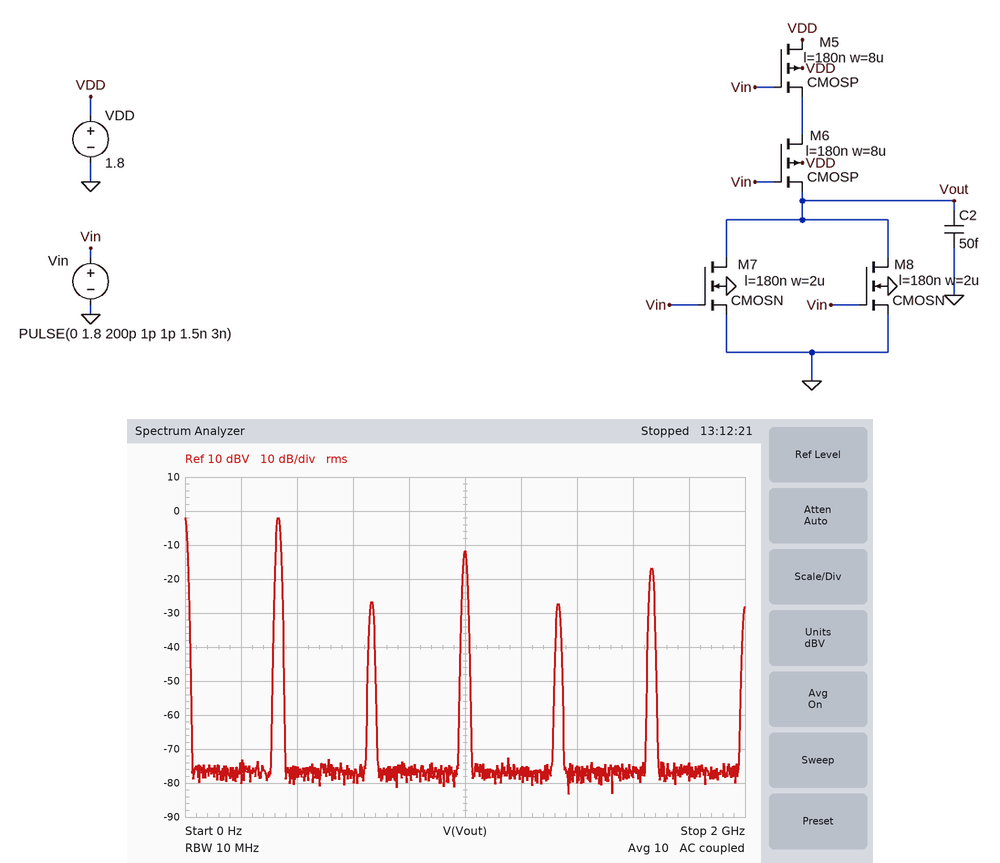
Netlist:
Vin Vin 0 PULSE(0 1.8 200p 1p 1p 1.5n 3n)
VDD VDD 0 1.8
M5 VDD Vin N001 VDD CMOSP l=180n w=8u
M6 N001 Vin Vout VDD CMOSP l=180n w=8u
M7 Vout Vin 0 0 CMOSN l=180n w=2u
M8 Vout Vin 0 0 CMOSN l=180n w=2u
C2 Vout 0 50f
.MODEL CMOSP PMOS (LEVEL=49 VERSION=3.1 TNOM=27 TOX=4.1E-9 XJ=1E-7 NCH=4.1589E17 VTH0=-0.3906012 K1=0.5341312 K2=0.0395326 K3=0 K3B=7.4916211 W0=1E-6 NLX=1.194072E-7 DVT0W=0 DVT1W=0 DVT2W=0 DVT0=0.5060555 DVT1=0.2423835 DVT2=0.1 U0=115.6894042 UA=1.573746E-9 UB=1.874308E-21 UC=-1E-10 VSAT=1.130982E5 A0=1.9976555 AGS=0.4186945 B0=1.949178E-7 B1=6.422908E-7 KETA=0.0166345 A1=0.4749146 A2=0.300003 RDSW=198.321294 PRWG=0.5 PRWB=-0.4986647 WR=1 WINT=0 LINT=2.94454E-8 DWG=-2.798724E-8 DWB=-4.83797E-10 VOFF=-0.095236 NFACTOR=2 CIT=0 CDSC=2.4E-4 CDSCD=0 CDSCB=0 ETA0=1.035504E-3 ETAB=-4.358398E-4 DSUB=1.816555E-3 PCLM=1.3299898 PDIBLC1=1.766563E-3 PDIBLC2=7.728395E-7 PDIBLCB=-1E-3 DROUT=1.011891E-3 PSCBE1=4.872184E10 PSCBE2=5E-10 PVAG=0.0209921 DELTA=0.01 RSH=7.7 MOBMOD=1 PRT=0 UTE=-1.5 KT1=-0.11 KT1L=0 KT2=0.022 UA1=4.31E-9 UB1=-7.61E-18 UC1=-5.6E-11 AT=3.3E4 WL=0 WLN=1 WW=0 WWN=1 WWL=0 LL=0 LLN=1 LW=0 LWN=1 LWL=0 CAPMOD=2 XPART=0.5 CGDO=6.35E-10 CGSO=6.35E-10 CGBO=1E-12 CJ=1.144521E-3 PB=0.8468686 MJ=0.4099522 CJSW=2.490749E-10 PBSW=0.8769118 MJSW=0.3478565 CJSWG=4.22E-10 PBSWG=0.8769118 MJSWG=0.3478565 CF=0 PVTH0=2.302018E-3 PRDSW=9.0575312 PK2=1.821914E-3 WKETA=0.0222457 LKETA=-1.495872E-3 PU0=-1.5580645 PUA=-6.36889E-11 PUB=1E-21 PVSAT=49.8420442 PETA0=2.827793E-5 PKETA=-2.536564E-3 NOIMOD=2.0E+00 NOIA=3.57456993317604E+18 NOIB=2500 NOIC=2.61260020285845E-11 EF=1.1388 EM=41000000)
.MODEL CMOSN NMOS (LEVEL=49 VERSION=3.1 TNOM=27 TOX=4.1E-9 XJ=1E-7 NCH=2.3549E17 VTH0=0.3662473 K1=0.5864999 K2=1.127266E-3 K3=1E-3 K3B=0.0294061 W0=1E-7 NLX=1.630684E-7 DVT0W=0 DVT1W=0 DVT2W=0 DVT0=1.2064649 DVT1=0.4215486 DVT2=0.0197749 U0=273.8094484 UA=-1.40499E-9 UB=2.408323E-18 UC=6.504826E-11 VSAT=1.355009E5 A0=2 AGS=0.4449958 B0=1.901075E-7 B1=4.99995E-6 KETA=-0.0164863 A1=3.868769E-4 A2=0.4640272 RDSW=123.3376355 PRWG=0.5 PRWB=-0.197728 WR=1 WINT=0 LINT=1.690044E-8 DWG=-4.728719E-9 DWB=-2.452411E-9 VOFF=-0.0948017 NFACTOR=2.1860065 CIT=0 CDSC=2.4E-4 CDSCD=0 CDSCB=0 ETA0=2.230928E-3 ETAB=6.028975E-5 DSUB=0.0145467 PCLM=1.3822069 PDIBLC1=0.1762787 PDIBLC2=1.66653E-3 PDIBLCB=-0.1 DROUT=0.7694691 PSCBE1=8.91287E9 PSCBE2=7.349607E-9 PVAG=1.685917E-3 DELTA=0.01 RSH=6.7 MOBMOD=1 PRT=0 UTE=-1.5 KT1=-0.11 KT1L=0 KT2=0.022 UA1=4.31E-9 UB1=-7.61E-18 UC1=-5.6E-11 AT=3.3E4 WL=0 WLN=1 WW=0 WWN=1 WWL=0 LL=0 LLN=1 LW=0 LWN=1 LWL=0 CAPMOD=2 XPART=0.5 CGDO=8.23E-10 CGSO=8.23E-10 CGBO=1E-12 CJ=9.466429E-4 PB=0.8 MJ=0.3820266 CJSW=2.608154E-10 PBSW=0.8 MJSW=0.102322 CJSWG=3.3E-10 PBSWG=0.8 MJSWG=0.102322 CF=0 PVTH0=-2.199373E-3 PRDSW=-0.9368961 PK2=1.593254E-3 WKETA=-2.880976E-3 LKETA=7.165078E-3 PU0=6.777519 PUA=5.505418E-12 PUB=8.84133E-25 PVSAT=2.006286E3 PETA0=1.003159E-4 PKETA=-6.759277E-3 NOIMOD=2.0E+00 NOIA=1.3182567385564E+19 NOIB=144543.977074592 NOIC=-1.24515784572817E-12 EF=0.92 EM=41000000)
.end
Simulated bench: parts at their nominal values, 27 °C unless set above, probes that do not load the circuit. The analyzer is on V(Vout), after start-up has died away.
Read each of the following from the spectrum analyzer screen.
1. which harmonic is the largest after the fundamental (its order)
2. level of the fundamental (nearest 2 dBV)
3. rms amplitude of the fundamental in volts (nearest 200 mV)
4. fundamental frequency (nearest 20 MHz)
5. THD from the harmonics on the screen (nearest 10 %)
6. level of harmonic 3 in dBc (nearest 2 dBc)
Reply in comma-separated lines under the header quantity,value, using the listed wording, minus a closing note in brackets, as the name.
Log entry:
quantity,value
which harmonic is the largest after the fundamental,3
level of the fundamental,-2 dBV
rms amplitude of the fundamental in volts,800 mV
fundamental frequency,340 MHz
THD from the harmonics on the screen,40 %
level of harmonic 3 in dBc,-10 dBc
